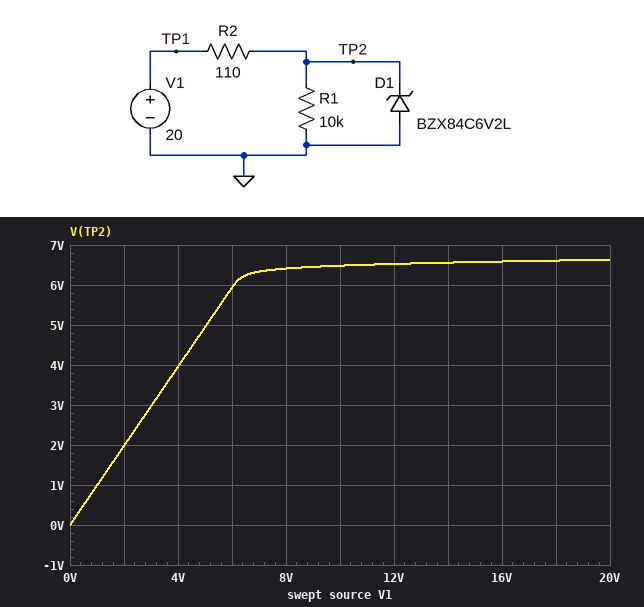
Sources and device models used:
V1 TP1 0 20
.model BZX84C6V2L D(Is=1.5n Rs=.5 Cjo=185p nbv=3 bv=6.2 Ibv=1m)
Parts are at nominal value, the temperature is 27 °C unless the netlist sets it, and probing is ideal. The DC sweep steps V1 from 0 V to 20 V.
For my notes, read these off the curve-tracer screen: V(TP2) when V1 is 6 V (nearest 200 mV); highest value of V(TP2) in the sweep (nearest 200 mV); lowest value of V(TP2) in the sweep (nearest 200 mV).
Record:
6.0 V
6.6 V
0 V
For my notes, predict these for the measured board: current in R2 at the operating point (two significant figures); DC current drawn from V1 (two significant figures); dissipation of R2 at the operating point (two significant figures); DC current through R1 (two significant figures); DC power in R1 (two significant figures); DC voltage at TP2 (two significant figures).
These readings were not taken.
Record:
120 mA
120 mA
1.6 W
660 µA
4.4 mW
6.6 V
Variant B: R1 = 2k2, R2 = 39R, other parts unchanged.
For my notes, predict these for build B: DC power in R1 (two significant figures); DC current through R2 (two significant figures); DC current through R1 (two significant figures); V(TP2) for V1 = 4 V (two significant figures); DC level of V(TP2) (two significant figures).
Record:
21 mW
340 mA
3.1 mA
3.9 V
6.8 V
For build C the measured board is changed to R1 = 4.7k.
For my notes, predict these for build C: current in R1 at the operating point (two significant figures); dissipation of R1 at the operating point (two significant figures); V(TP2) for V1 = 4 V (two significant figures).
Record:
1.4 mA
9.4 mW
3.9 V
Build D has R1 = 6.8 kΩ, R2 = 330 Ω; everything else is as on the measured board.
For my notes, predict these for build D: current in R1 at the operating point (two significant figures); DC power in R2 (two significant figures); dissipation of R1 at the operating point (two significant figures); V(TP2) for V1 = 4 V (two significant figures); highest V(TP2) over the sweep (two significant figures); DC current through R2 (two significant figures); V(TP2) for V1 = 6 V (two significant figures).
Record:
960 µA
550 mW
6.2 mW
3.8 V
6.5 V
41 mA
5.7 V
